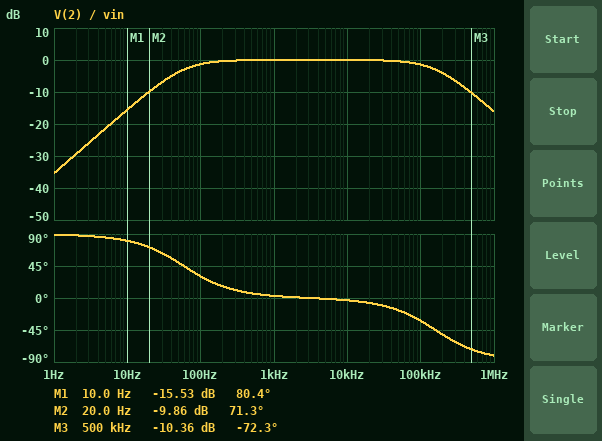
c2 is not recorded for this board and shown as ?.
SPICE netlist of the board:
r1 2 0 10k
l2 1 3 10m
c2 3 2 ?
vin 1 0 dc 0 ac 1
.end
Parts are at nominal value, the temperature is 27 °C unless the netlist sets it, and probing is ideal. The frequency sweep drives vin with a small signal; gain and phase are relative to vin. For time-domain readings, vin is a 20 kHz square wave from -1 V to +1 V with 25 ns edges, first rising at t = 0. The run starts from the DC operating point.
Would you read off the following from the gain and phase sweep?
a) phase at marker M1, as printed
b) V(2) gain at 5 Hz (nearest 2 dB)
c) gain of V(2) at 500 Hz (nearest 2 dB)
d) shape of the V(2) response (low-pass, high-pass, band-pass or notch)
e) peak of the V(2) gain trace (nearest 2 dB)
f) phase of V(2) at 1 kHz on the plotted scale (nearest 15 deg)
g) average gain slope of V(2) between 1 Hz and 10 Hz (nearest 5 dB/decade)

80.4 deg
-22 dB
0 dB
band-pass
0 dB
0 deg
20 dB/decade
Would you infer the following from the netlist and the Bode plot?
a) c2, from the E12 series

270 nF
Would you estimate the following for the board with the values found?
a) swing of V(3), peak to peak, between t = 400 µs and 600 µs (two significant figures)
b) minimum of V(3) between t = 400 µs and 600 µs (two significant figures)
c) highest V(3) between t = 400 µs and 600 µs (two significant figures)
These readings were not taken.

2.0 V
-1.0 V
1.0 V
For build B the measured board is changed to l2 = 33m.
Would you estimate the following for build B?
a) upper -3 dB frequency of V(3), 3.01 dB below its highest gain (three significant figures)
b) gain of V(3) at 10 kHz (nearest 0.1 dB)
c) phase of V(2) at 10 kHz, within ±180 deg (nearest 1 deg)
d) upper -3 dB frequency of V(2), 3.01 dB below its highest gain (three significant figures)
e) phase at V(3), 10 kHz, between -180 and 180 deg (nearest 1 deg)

48.2 kHz
-0.2 dB
-11 deg
48.3 kHz
-12 deg
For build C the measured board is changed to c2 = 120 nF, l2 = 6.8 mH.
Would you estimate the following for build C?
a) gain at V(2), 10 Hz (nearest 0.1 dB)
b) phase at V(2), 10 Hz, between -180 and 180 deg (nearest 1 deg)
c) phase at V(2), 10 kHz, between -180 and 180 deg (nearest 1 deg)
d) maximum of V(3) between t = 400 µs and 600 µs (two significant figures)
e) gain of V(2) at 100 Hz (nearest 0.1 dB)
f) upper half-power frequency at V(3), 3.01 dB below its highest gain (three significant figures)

-22.5 dB
86 deg
-2 deg
1.0 V
-4.4 dB
234 kHz
